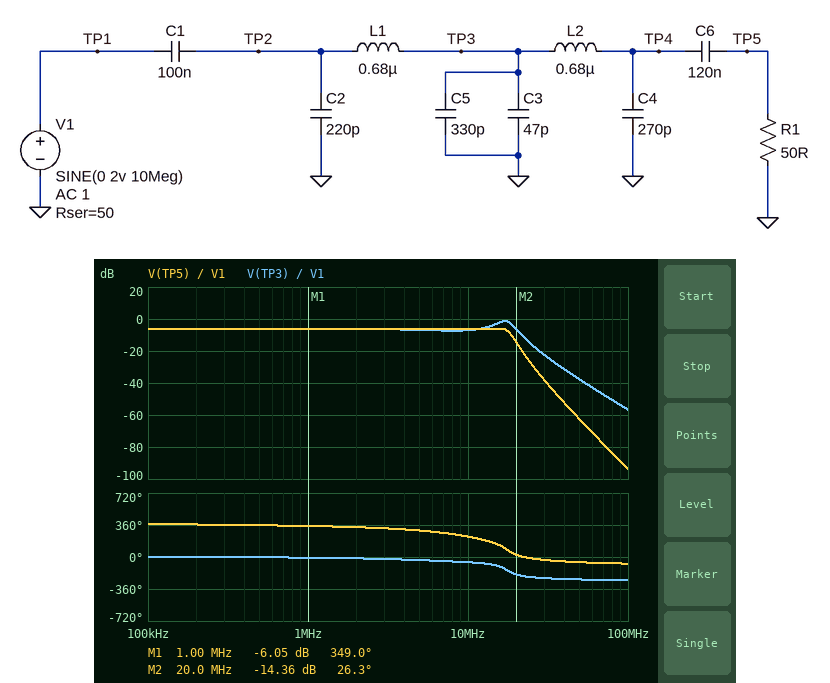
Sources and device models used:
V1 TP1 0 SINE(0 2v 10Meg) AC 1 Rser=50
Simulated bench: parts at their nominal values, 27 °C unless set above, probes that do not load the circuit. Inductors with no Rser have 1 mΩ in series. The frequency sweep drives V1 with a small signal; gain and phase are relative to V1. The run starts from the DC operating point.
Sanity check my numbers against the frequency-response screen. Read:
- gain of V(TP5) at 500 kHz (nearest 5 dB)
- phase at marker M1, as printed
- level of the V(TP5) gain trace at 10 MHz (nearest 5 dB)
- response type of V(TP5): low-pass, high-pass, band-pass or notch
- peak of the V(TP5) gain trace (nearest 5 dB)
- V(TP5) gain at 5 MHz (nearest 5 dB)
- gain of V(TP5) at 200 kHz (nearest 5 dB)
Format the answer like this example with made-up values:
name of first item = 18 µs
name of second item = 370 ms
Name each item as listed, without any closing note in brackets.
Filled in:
gain of V(TP5) at 500 kHz = -5 dB
phase at marker M1, as printed = 349.0 deg
level of the V(TP5) gain trace at 10 MHz = -5 dB
response type of V(TP5): low-pass, high-pass, band-pass or notch = low-pass
peak of the V(TP5) gain trace = -5 dB
V(TP5) gain at 5 MHz = -5 dB
gain of V(TP5) at 200 kHz = -5 dB
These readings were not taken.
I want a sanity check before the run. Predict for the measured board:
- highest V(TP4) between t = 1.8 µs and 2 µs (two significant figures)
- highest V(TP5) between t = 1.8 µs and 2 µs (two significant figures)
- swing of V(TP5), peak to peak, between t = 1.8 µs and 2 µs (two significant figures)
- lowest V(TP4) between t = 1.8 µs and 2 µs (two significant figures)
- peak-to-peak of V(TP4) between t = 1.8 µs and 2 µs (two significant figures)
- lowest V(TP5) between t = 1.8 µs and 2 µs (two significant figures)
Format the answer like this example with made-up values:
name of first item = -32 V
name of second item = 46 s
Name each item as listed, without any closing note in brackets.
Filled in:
highest V(TP4) between t = 1.8 µs and 2 µs = 990 mV
highest V(TP5) between t = 1.8 µs and 2 µs = 990 mV
swing of V(TP5), peak to peak, between t = 1.8 µs and 2 µs = 2.0 V
lowest V(TP4) between t = 1.8 µs and 2 µs = -990 mV
peak-to-peak of V(TP4) between t = 1.8 µs and 2 µs = 2.0 V
lowest V(TP5) between t = 1.8 µs and 2 µs = -1.0 V
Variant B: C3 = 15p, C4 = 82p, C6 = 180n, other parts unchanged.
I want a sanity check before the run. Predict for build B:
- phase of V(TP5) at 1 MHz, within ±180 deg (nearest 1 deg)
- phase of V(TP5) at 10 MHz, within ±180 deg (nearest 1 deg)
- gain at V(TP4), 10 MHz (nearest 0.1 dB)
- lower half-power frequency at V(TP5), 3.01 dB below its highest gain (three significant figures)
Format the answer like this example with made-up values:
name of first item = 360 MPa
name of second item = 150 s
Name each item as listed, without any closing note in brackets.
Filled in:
phase of V(TP5) at 1 MHz, within ±180 deg = -9 deg
phase of V(TP5) at 10 MHz, within ±180 deg = -111 deg
gain at V(TP4), 10 MHz = -6.2 dB
lower half-power frequency at V(TP5), 3.01 dB below its highest gain = 24.8 kHz
